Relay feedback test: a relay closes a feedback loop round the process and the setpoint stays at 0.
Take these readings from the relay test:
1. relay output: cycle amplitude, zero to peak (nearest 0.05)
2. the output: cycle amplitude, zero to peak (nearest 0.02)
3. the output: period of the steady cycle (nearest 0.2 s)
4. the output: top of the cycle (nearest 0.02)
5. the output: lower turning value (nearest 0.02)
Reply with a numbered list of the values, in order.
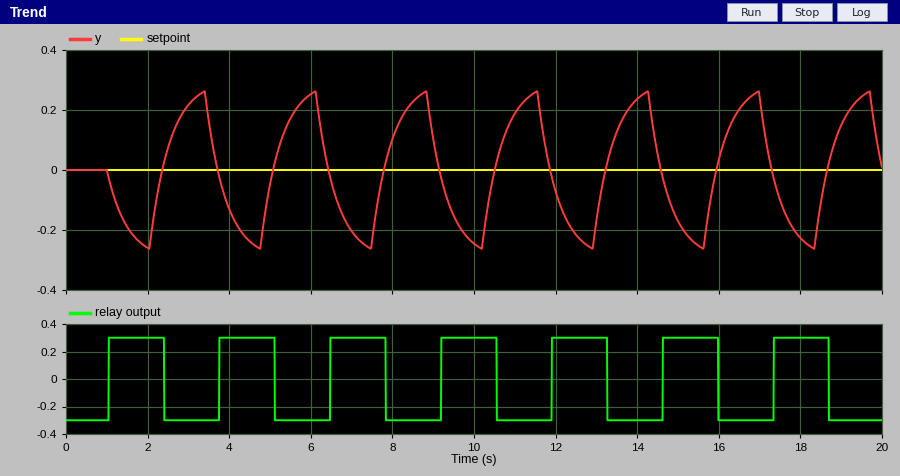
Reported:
1. 0.30
2. 0.26
3. 2.8 s
4. 0.26
5. -0.26
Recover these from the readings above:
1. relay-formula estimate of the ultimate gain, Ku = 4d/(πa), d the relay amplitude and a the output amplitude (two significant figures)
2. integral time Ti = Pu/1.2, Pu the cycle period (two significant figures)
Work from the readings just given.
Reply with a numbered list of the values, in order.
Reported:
1. 1.5
2. 2.3 s
